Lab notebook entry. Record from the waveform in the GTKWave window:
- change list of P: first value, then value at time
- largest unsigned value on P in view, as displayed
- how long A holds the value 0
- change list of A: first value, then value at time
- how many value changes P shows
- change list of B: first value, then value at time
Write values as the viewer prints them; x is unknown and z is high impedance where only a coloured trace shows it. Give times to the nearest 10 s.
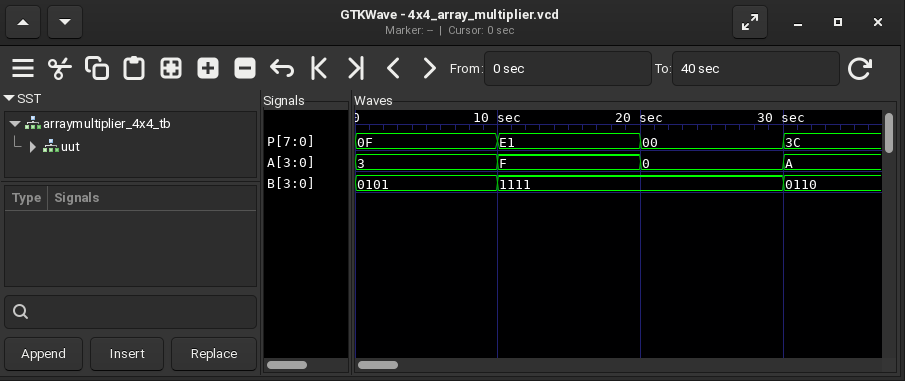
0F, E1 at 10 s, 00 at 20 s, 3C at 30 s
E1
10 s
3, F at 10 s, 0 at 20 s, A at 30 s
3
0101, 1111 at 10 s, 0110 at 30 s
